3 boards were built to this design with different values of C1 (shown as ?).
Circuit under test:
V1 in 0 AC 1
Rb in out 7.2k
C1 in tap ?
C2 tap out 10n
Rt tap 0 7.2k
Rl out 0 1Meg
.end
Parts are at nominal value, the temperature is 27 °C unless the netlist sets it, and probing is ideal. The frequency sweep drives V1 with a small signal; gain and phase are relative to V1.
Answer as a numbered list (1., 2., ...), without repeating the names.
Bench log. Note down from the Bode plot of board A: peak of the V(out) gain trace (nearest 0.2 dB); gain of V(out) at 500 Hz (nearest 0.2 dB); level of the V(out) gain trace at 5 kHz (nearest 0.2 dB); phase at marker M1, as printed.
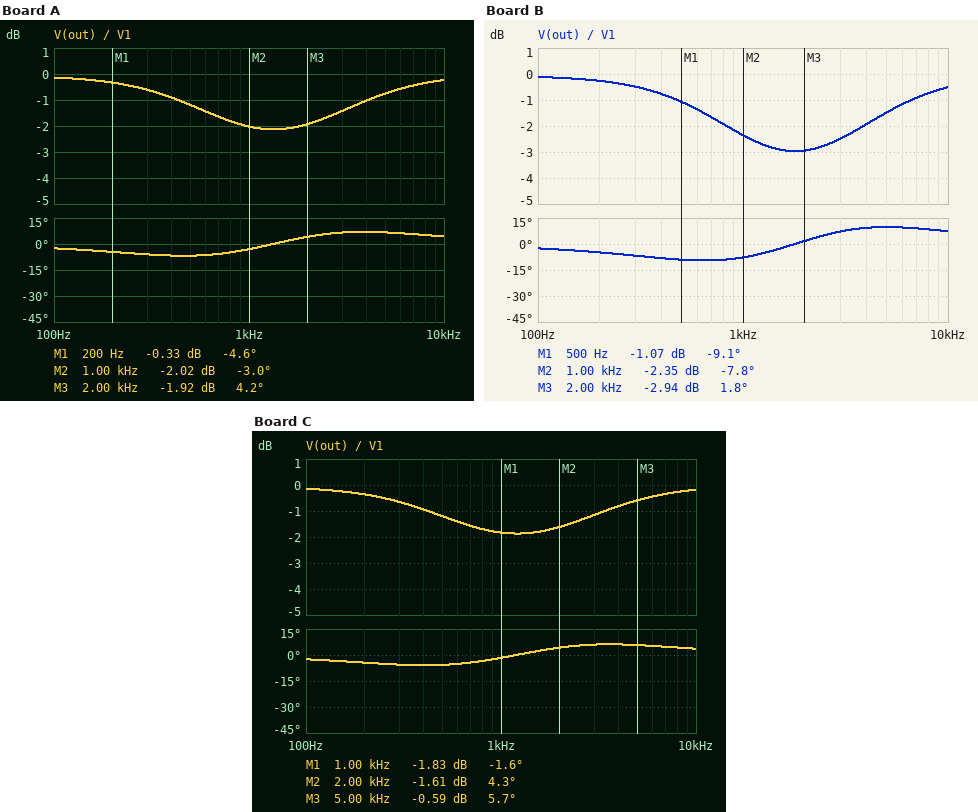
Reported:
1. -0.2 dB
2. -1.2 dB
3. -0.8 dB
4. -4.6 deg
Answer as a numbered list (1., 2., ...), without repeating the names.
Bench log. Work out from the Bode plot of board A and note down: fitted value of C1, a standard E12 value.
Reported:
1. 27 nF
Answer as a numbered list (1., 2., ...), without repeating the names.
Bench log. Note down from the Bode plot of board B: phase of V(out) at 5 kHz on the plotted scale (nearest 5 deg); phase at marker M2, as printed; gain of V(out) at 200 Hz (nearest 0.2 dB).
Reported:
1. 10 deg
2. -7.8 deg
3. -0.2 dB
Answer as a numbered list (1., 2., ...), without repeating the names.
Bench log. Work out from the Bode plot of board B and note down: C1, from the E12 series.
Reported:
1. 15 nF
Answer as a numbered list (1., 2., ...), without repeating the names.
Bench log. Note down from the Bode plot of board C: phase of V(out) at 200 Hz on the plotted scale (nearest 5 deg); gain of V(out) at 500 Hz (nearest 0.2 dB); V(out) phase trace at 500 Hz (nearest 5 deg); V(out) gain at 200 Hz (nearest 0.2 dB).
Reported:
1. -5 deg
2. -1.2 dB
3. -5 deg
4. -0.4 dB
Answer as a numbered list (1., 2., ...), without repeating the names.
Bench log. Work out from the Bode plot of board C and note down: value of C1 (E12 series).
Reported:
1. 33 nF
